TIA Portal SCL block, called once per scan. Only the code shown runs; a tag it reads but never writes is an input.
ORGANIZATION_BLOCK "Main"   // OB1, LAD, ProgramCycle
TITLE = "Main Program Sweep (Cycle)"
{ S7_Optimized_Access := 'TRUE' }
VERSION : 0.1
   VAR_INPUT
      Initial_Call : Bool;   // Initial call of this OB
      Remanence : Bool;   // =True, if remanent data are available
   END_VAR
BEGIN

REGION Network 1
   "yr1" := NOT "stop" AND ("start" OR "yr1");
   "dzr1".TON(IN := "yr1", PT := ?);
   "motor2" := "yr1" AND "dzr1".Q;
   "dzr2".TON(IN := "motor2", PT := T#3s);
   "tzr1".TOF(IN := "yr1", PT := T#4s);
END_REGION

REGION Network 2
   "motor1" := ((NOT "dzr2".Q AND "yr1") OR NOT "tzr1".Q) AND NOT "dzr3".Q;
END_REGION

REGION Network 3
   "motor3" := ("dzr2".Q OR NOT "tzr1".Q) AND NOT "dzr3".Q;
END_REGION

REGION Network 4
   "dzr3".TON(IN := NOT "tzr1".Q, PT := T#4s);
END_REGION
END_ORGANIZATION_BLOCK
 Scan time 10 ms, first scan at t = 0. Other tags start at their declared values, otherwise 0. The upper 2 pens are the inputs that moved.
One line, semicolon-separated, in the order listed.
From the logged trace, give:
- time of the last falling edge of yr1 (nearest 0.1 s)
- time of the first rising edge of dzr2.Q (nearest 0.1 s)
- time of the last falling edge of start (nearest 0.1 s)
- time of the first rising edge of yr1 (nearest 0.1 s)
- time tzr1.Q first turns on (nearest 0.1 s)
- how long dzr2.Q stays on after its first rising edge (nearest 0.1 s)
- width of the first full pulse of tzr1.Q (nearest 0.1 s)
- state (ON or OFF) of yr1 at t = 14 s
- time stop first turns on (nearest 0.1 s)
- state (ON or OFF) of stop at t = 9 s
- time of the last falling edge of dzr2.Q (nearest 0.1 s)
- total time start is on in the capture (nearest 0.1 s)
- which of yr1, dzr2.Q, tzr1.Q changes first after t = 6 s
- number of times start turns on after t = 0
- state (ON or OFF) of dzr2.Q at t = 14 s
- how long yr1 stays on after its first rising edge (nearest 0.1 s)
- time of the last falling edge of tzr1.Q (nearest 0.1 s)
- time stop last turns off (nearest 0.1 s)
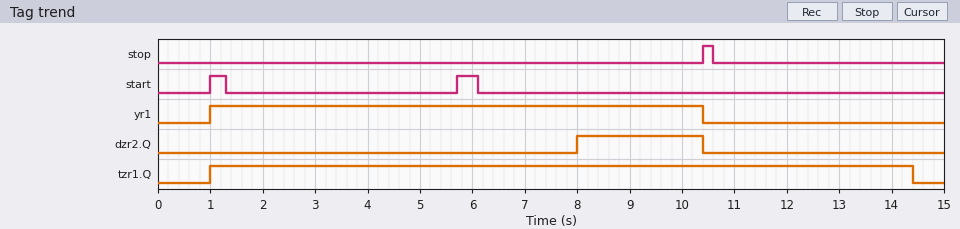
10.4 s; 8.0 s; 6.1 s; 1.0 s; 1.0 s; 2.4 s; 13.4 s; OFF; 10.4 s; OFF; 10.4 s; 0.7 s; dzr2.Q; 2; OFF; 9.4 s; 14.4 s; 10.6 s
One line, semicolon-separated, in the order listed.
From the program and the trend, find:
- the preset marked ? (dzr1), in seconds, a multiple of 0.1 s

4.0 s
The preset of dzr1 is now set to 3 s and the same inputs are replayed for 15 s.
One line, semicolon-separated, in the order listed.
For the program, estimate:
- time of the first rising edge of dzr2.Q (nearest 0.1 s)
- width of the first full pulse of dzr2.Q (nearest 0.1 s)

7.0 s; 3.4 s
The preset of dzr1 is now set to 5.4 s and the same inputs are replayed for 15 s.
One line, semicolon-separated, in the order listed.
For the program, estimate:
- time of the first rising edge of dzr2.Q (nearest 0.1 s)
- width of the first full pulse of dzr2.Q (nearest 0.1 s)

9.4 s; 1.0 s
